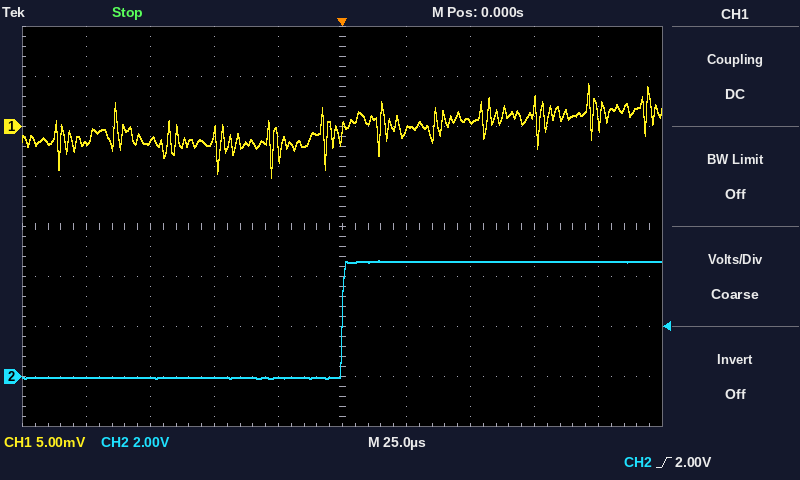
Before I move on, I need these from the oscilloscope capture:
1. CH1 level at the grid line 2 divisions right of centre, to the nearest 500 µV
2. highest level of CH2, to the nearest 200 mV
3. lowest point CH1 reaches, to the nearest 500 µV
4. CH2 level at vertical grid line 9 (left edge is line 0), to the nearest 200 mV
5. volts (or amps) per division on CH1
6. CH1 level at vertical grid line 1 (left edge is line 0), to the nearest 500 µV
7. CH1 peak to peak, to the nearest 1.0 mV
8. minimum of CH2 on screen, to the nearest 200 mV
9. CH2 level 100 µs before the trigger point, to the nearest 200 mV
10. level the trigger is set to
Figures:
500 µV
4.6 V
-5.0 mV
4.6 V
5 mV
-1.5 mV
9.0 mV
0.0 V
0.0 V
2.00 V
